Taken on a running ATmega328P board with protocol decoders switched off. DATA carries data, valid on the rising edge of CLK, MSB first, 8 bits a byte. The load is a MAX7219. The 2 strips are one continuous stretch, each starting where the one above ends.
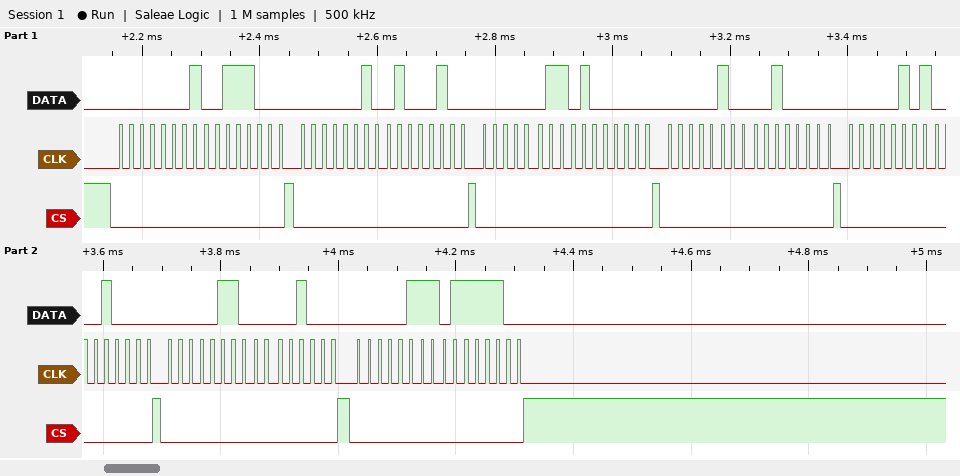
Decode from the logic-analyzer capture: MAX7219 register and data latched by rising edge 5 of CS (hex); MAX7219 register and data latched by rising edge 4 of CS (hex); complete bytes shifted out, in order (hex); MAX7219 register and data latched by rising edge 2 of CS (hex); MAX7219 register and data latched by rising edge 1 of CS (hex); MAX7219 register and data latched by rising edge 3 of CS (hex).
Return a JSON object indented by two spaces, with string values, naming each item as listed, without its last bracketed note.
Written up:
{
  "MAX7219 register and data latched by rising edge 5 of CS": "register 0x5, data 0x10",
  "MAX7219 register and data latched by rising edge 4 of CS": "register 0x4, data 0x20",
  "complete bytes shifted out, in order": "01 38 02 44 03 40 04 20 05 10 06 08 07 7C",
  "MAX7219 register and data latched by rising edge 2 of CS": "register 0x2, data 0x44",
  "MAX7219 register and data latched by rising edge 1 of CS": "register 0x1, data 0x38",
  "MAX7219 register and data latched by rising edge 3 of CS": "register 0x3, data 0x40"
}
